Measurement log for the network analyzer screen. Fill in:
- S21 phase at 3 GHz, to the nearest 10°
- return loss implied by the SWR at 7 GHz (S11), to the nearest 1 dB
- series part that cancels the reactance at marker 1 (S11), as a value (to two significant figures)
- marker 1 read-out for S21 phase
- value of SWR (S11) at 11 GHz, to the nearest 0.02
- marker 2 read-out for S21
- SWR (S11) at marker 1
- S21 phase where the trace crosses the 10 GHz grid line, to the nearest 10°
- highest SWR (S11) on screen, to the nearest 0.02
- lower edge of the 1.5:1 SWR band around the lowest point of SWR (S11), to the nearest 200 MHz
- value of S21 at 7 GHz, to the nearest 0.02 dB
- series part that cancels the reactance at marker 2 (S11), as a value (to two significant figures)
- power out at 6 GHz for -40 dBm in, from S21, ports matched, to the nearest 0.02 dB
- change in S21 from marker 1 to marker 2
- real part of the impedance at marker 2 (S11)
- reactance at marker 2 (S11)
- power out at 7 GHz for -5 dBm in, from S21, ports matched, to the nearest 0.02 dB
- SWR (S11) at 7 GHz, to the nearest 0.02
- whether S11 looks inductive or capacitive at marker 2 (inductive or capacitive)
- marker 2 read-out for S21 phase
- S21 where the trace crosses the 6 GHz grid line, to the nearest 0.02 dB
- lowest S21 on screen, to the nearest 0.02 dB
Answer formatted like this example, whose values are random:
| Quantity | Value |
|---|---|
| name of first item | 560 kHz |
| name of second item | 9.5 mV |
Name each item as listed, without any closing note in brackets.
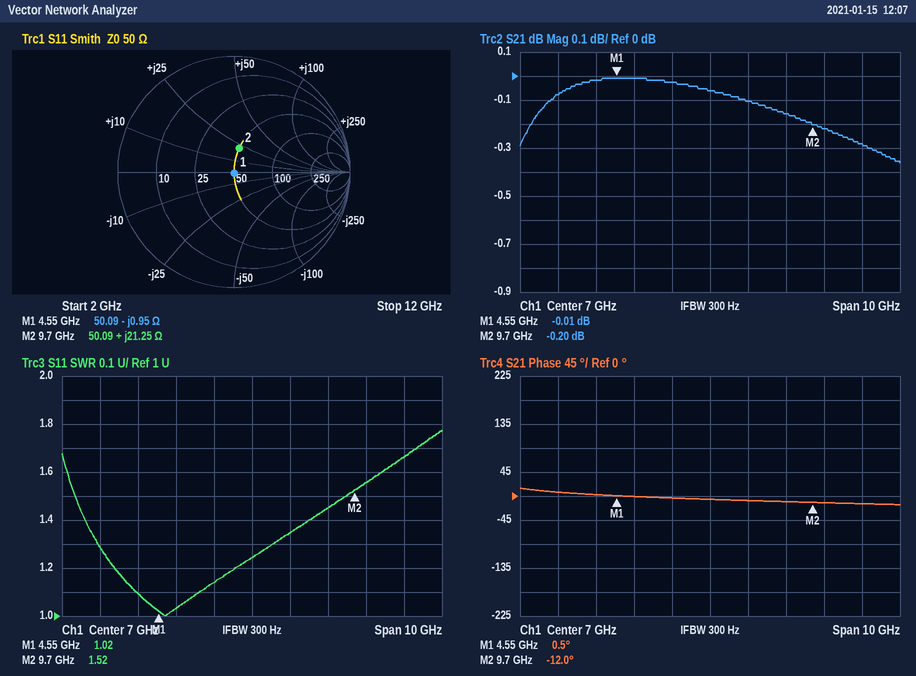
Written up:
| Quantity | Value |
|---|---|
| S21 phase at 3 GHz, to the nearest 10° | 10° |
| return loss implied by the SWR at 7 GHz (S11), to the nearest 1 dB | 19 dB |
| series part that cancels the reactance at marker 1 (S11), as a value | 33 pH |
| marker 1 read-out for S21 phase | 0.5° |
| value of SWR (S11) at 11 GHz, to the nearest 0.02 | 1.66 |
| marker 2 read-out for S21 | -0.20 dB |
| SWR (S11) at marker 1 | 1.02 |
| S21 phase where the trace crosses the 10 GHz grid line, to the nearest 10° | -10° |
| highest SWR (S11) on screen, to the nearest 0.02 | 1.78 |
| lower edge of the 1.5:1 SWR band around the lowest point of SWR (S11), to the nearest 200 MHz | 2.4 GHz |
| value of S21 at 7 GHz, to the nearest 0.02 dB | -0.06 dB |
| series part that cancels the reactance at marker 2 (S11), as a value | 770 fF |
| power out at 6 GHz for -40 dBm in, from S21, ports matched, to the nearest 0.02 dB | -40.02 dBm |
| change in S21 from marker 1 to marker 2 | -0.19 dB |
| real part of the impedance at marker 2 | 50.09 Ω |
| reactance at marker 2 | +21.25 Ω |
| power out at 7 GHz for -5 dBm in, from S21, ports matched, to the nearest 0.02 dB | -5.06 dBm |
| SWR (S11) at 7 GHz, to the nearest 0.02 | 1.24 |
| whether S11 looks inductive or capacitive at marker 2 | inductive |
| marker 2 read-out for S21 phase | -12.0° |
| S21 where the trace crosses the 6 GHz grid line, to the nearest 0.02 dB | -0.02 dB |
| lowest S21 on screen, to the nearest 0.02 dB | -0.36 dB |
